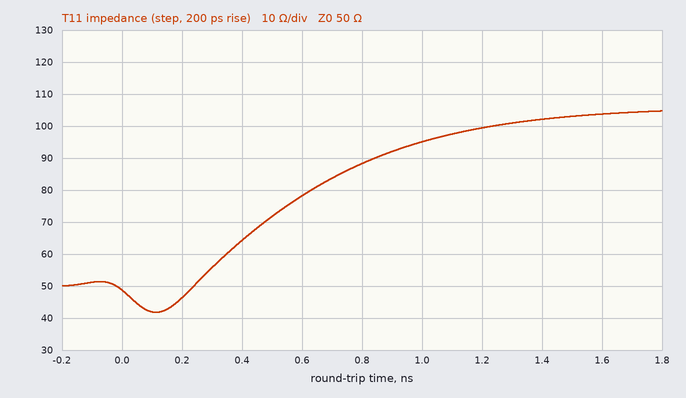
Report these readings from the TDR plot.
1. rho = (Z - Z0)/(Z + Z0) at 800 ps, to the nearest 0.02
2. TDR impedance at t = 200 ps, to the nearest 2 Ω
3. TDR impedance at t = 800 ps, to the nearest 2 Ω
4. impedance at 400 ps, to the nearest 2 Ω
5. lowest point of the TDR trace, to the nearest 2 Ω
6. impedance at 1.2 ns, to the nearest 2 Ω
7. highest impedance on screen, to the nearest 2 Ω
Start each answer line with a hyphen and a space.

- +0.28
- 46 Ω
- 88 Ω
- 64 Ω
- 42 Ω
- 100 Ω
- 104 Ω
